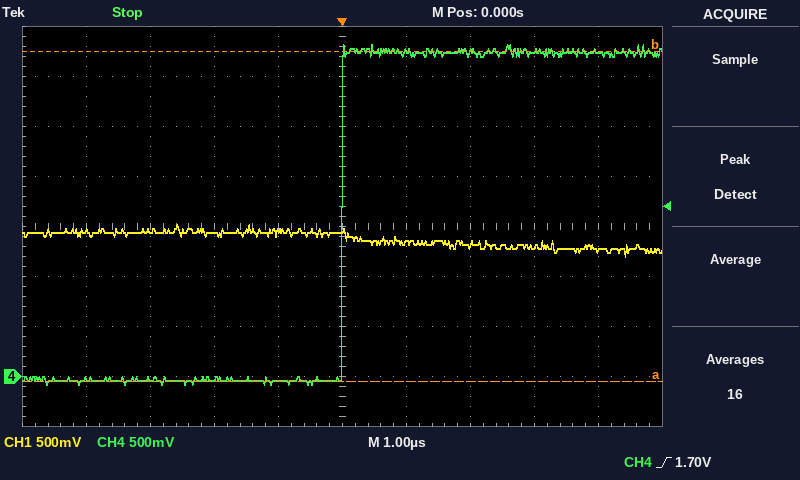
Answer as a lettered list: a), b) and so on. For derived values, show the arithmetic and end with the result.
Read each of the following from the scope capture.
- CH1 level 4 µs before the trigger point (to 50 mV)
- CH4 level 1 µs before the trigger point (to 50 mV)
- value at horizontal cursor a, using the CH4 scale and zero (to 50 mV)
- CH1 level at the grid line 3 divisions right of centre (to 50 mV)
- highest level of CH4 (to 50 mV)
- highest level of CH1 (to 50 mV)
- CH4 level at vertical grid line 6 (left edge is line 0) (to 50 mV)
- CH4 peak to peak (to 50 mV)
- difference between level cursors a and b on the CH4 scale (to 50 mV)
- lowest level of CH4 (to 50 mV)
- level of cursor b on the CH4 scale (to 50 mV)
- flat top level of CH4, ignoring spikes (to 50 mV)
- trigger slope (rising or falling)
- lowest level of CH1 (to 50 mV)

a) 1.45 V
b) -50 mV
c) -50 mV
d) 1.30 V
e) 3.30 V
f) 1.50 V
g) 3.25 V
h) 3.30 V − (-100 mV) = 3.40 V
i) 3.30 V
j) -100 mV
k) 3.25 V
l) 3.25 V
m) rising
n) 1.20 V
